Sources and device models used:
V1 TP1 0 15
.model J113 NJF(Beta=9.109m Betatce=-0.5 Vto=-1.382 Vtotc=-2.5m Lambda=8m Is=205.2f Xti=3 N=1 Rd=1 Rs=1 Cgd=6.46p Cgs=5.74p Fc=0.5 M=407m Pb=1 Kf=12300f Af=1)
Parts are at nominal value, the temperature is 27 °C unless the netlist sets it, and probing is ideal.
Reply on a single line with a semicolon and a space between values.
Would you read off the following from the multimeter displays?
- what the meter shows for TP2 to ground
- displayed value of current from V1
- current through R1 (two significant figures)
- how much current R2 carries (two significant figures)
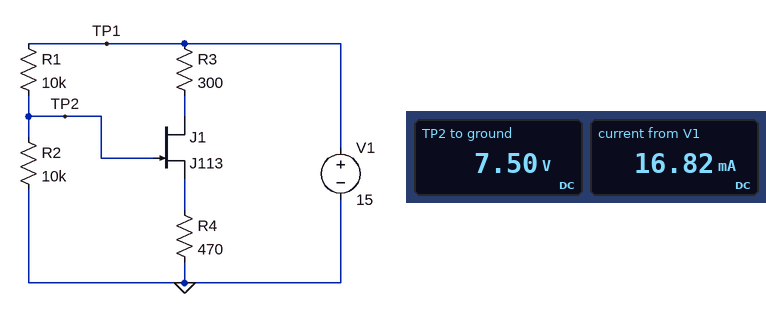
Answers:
7.50 V; 16.82 mA; 750 µA; 750 µA
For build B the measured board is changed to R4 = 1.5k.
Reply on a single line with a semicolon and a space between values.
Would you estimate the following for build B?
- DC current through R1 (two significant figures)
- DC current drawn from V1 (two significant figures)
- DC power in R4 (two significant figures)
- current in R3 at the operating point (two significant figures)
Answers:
750 µA; 6.2 mA; 44 mW; 5.4 mA
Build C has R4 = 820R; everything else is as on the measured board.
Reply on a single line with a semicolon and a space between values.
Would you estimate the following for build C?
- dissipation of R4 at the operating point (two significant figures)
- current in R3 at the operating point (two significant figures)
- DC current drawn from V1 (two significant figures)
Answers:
75 mW; 9.6 mA; 10 mA
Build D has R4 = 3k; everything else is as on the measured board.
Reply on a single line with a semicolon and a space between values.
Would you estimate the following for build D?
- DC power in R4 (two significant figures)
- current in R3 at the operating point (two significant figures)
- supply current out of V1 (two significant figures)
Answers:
23 mW; 2.8 mA; 3.5 mA
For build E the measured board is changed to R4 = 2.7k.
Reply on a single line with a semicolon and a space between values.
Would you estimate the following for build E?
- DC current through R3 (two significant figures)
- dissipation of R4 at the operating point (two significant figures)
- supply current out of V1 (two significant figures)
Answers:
3.1 mA; 26 mW; 3.8 mA
